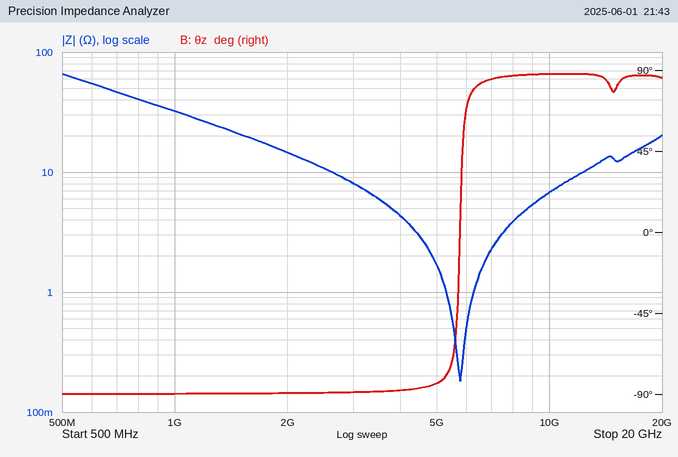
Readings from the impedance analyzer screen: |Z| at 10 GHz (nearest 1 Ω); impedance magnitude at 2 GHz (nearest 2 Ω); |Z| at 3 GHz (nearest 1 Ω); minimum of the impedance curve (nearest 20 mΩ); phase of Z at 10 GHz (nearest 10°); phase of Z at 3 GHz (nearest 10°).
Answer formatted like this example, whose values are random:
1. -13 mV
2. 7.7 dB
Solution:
1. 7 Ω
2. 14 Ω
3. 8 Ω
4. 180 mΩ
5. 90°
6. -90°
